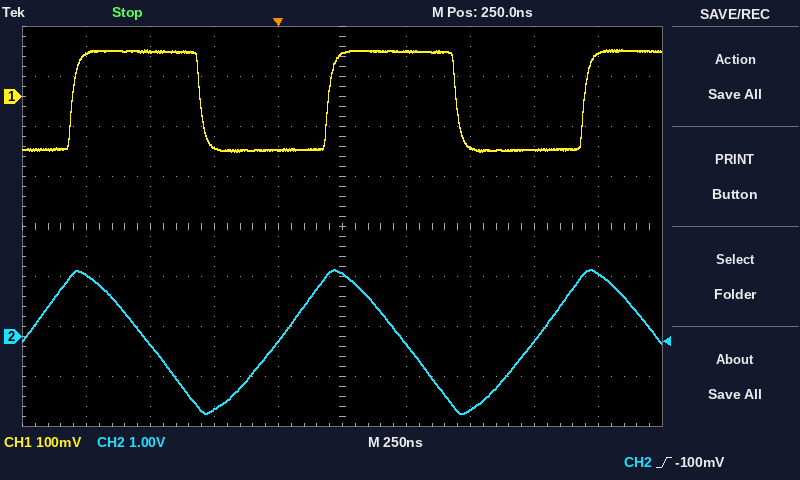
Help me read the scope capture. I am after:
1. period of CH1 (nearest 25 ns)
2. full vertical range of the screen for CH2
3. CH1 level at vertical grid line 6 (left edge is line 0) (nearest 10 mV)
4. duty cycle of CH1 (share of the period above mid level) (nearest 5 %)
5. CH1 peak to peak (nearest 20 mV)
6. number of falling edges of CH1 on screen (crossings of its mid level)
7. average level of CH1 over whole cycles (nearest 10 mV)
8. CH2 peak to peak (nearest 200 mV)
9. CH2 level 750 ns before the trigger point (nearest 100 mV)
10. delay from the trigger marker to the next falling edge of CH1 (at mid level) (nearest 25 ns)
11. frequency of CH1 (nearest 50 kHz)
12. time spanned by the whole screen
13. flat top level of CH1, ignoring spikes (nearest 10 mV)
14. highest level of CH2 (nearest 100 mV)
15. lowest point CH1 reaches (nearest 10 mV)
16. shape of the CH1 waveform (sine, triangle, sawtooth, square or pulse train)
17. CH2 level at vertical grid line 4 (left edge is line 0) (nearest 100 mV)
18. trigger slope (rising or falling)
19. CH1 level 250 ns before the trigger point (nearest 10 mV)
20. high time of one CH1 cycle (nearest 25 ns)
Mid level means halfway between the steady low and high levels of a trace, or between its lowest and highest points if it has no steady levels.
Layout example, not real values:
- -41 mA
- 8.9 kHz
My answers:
- 1.000 µs
- 8 V
- 90 mV
- 50 %
- 200 mV
- 2
- -10 mV
- 2.8 V
- 1.2 V
- 700 ns
- 1.00 MHz
- 2.5 µs
- 90 mV
- 1.3 V
- -110 mV
- square
- -100 mV
- rising
- -100 mV
- 500 ns
